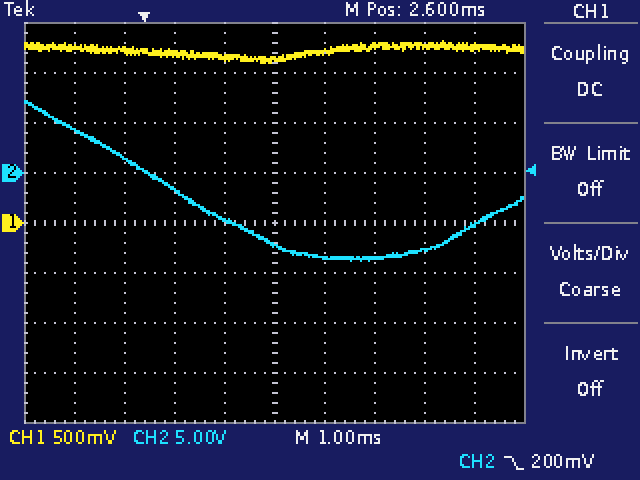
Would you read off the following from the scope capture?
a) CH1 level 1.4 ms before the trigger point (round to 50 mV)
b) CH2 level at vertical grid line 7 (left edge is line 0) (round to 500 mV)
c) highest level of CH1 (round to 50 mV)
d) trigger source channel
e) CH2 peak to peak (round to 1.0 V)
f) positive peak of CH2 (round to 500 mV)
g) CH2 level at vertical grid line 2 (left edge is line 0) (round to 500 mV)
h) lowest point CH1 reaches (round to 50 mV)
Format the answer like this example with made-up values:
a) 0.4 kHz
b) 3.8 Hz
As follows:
a) 1.75 V
b) -8.5 V
c) 1.80 V
d) CH2
e) 16.0 V
f) 7.0 V
g) 1.5 V
h) 1.60 V
